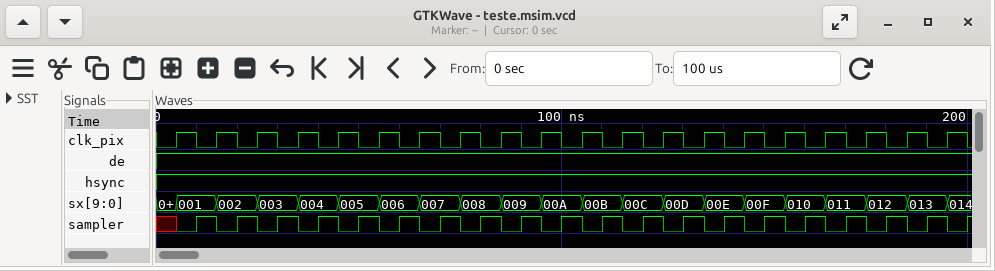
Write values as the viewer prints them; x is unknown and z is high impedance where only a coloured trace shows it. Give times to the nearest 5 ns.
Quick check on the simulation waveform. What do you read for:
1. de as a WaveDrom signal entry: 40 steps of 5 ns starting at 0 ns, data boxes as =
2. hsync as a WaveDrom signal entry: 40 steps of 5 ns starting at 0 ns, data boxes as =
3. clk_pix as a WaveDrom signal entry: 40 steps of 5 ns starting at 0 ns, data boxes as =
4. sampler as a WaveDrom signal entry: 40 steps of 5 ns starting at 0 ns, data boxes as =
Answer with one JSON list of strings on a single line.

["{name: 'de', wave: '1.......................................'}", "{name: 'hsync', wave: '1.......................................'}", "{name: 'clk_pix', wave: '0101010101010101010101010101010101010101'}", "{name: 'sampler', wave: 'x010101010101010101010101010101010101010'}"]
